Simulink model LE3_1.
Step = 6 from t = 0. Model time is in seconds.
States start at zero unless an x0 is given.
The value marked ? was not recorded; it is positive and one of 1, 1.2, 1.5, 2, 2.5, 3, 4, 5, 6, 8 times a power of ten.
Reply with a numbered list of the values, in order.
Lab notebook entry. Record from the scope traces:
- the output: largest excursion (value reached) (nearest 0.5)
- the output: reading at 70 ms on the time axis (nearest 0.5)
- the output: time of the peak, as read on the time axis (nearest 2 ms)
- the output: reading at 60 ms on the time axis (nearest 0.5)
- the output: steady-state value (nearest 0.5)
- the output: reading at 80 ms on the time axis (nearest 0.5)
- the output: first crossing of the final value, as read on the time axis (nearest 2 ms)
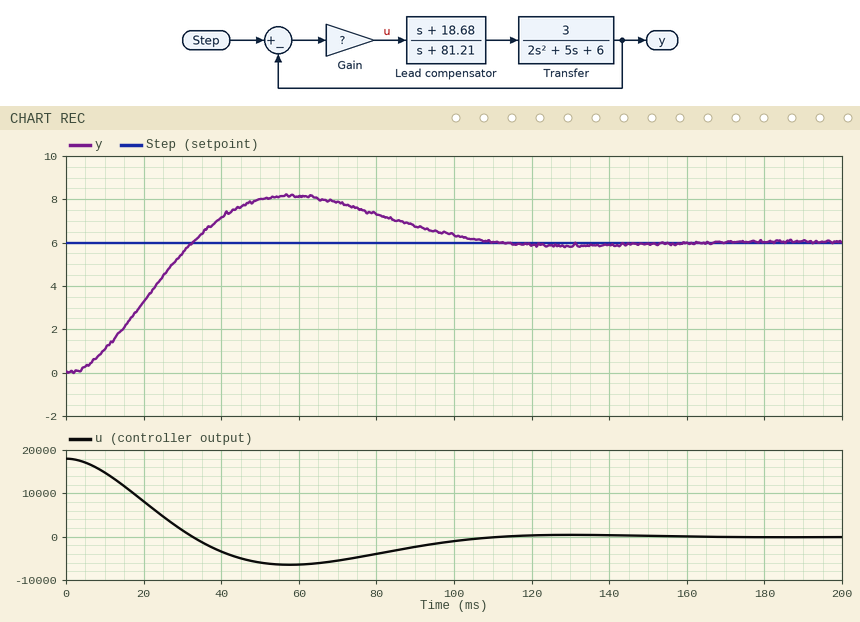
1. 8.0
2. 8.0
3. 58 ms
4. 8.0
5. 6.0
6. 7.5
7. 32 ms
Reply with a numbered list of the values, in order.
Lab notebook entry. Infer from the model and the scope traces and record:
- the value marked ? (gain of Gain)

1. 3000
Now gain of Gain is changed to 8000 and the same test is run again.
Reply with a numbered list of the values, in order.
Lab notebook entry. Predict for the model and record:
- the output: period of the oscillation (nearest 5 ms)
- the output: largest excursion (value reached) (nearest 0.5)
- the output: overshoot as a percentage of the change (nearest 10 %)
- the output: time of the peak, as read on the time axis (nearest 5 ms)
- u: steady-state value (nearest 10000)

1. 65 ms
2. 9.0
3. 50 %
4. 30 ms
5. 0
